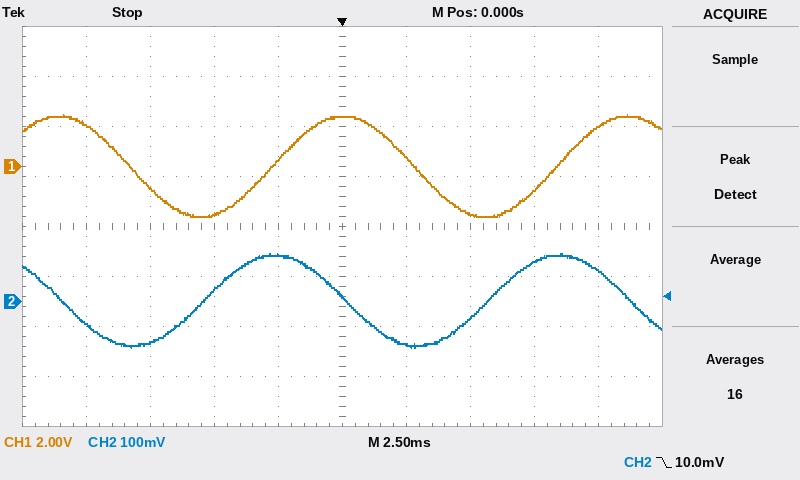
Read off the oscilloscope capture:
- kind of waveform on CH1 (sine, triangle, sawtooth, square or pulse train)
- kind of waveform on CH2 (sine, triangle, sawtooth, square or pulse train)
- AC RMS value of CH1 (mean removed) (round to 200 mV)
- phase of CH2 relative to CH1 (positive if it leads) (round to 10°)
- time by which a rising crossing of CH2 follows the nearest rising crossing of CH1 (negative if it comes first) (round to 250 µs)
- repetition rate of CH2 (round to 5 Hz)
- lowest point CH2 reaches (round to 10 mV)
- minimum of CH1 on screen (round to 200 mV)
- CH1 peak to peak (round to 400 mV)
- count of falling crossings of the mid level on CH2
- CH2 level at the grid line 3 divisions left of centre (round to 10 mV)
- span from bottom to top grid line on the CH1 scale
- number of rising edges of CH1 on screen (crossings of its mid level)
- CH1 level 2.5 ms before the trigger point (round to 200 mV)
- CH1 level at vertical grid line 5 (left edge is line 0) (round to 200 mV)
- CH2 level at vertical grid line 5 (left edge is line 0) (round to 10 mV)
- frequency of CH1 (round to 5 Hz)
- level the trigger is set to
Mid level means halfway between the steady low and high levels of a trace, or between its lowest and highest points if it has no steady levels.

sine
sine
1.4 V
+90°
-2.75 ms
90 Hz
-90 mV
-2.0 V
4.0 V
3
-80 mV
16 V
2
200 mV
2.0 V
10 mV
90 Hz
10.0 mV
